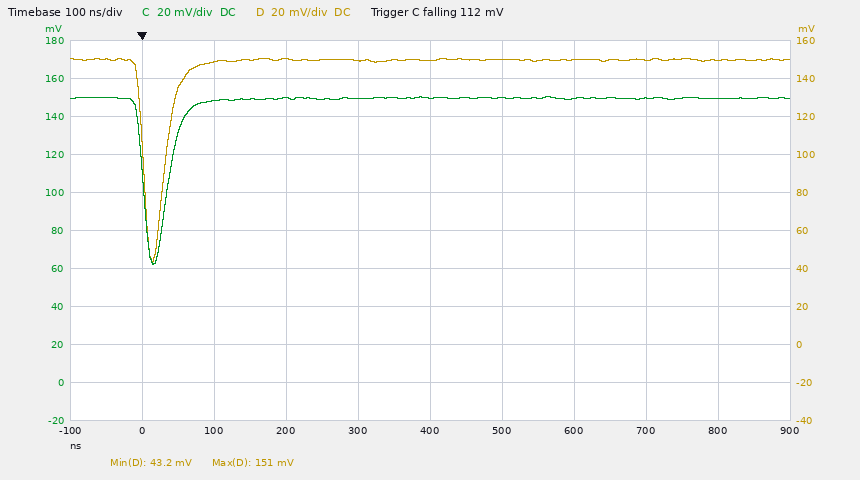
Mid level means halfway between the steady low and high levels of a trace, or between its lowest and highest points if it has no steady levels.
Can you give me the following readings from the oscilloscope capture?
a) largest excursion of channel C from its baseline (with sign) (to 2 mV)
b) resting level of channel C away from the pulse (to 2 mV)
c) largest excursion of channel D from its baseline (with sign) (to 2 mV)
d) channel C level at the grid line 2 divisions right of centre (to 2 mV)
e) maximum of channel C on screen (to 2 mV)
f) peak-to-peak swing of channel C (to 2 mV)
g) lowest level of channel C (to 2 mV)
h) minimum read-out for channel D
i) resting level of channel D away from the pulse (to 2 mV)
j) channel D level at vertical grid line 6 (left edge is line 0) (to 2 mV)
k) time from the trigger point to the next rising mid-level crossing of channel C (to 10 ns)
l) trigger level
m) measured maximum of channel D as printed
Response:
-88 mV
150 mV
-106 mV
150 mV
150 mV
88 mV
62 mV
43.2 mV
150 mV
150 mV
40 ns
112 mV
151 mV
